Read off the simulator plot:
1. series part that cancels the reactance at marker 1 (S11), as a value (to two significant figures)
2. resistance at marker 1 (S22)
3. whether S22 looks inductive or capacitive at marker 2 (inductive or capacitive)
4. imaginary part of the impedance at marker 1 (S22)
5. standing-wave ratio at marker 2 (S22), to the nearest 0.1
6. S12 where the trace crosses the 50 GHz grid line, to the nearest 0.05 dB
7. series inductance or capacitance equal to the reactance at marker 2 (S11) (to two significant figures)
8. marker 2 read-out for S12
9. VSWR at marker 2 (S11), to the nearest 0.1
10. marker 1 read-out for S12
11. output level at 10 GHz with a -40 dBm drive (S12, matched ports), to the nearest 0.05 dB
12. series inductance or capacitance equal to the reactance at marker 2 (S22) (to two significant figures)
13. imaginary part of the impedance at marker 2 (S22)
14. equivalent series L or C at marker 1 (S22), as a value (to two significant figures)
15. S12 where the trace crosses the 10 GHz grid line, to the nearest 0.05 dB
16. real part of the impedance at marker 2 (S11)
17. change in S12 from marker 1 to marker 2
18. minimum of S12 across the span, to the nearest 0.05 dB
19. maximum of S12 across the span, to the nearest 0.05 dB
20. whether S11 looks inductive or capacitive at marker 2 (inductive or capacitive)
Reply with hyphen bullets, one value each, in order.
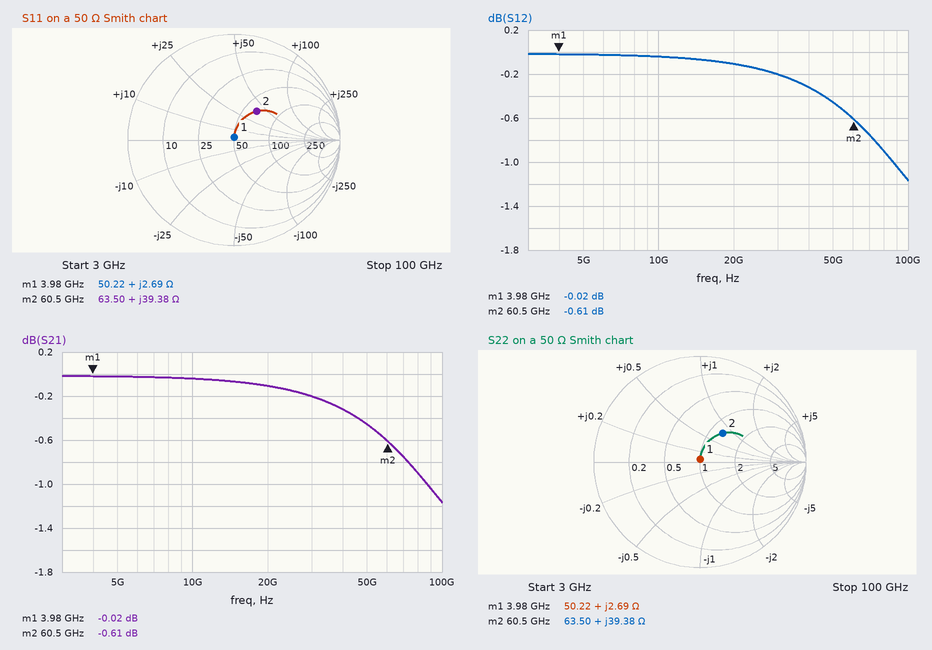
- 15 pF
- 50.22 Ω
- inductive
- +2.69 Ω
- 2.1
- -0.45 dB
- 100 pH
- -0.61 dB
- 2.1
- -0.02 dB
- -40.05 dBm
- 100 pH
- +39.38 Ω
- 110 pH
- -0.05 dB
- 63.50 Ω
- -0.59 dB
- -1.15 dB
- 0.00 dB
- inductive
